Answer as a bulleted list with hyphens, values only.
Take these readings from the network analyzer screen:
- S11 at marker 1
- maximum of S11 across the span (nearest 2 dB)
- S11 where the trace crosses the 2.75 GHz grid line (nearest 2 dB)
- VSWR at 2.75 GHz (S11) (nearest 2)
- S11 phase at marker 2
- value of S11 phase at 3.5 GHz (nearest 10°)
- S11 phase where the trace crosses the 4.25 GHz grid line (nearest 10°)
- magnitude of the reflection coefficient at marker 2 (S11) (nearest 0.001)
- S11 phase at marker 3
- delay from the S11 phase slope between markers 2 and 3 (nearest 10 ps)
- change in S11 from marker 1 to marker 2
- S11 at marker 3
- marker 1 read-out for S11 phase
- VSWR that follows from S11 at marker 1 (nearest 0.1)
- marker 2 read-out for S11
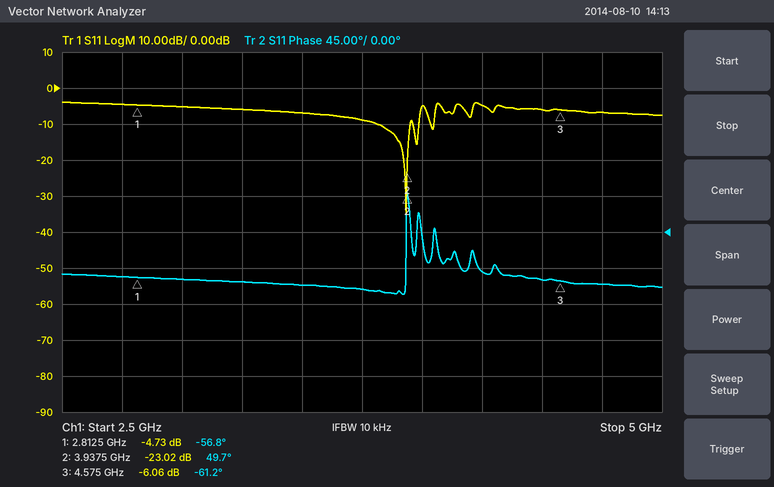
- -4.73 dB
- -4 dB
- -4 dB
- 4
- 49.7°
- -70°
- -50°
- 0.071
- -61.2°
- 480 ps
- -18.29 dB
- -6.06 dB
- -56.8°
- 3.8
- -23.02 dB
